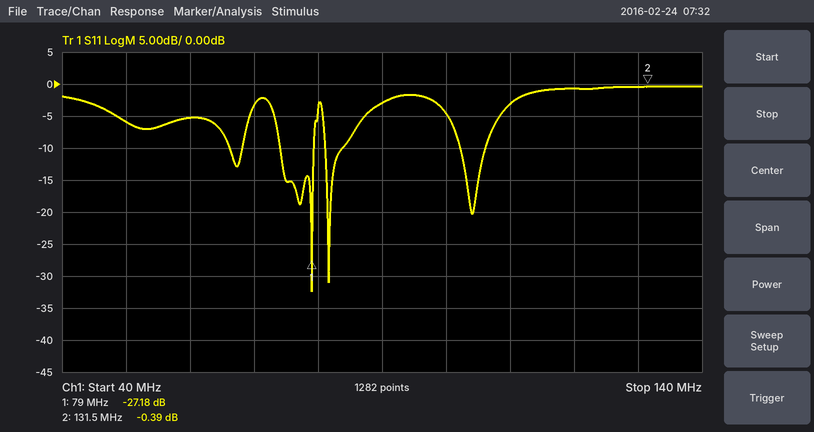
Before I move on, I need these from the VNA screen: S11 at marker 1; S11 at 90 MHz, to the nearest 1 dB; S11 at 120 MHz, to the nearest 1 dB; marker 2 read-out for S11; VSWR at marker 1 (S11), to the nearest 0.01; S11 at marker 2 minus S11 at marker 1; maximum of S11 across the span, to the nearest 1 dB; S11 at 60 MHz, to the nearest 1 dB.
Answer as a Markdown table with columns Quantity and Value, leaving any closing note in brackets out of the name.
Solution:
| Quantity | Value |
|---|---|
| S11 at marker 1 | -27.18 dB |
| S11 at 90 MHz, to the nearest 1 dB | -3 dB |
| S11 at 120 MHz, to the nearest 1 dB | -1 dB |
| marker 2 read-out for S11 | -0.39 dB |
| VSWR at marker 1 (S11), to the nearest 0.01 | 1.09 |
| S11 at marker 2 minus S11 at marker 1 | 26.79 dB |
| maximum of S11 across the span, to the nearest 1 dB | 0 dB |
| S11 at 60 MHz, to the nearest 1 dB | -5 dB |
